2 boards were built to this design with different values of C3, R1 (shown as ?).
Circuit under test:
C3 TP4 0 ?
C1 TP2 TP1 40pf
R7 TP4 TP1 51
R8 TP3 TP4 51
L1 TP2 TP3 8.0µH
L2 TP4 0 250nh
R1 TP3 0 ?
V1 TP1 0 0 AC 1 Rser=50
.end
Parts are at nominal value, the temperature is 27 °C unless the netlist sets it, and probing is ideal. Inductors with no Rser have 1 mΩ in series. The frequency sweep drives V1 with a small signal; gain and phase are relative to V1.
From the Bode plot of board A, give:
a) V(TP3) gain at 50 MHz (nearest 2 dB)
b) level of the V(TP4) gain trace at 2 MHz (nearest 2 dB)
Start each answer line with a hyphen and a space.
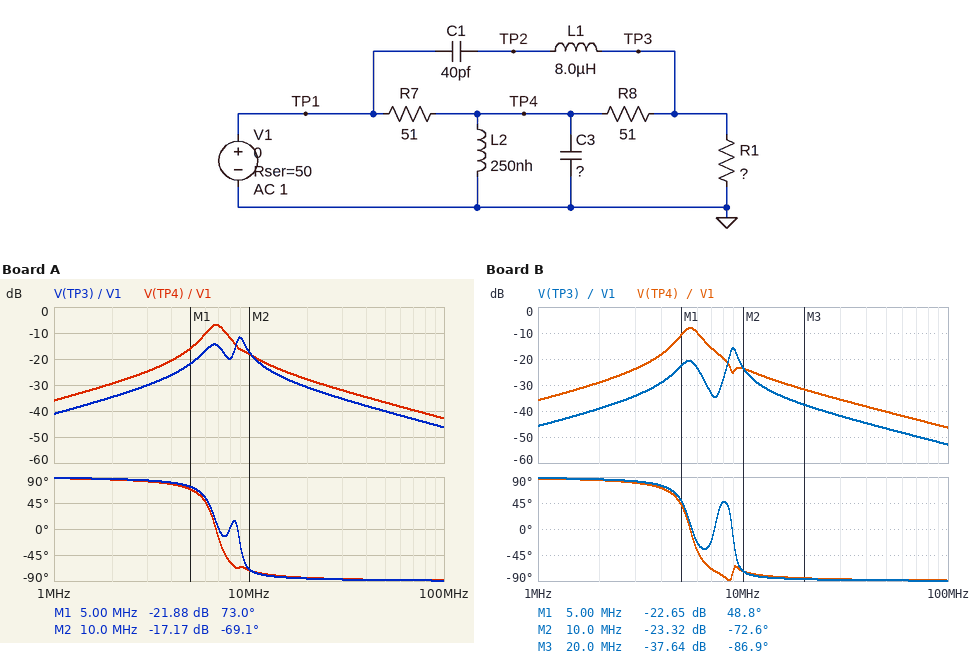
- -40 dB
- -30 dB
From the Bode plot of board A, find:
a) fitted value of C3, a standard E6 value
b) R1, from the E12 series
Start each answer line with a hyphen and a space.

- 2.2 nF
- 33 Ω
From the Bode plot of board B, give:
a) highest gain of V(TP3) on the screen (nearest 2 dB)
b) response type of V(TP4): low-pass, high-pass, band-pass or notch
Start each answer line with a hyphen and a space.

- -16 dB
- band-pass
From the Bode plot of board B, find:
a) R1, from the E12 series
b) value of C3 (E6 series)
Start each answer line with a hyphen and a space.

- 15 Ω
- 3.3 nF
